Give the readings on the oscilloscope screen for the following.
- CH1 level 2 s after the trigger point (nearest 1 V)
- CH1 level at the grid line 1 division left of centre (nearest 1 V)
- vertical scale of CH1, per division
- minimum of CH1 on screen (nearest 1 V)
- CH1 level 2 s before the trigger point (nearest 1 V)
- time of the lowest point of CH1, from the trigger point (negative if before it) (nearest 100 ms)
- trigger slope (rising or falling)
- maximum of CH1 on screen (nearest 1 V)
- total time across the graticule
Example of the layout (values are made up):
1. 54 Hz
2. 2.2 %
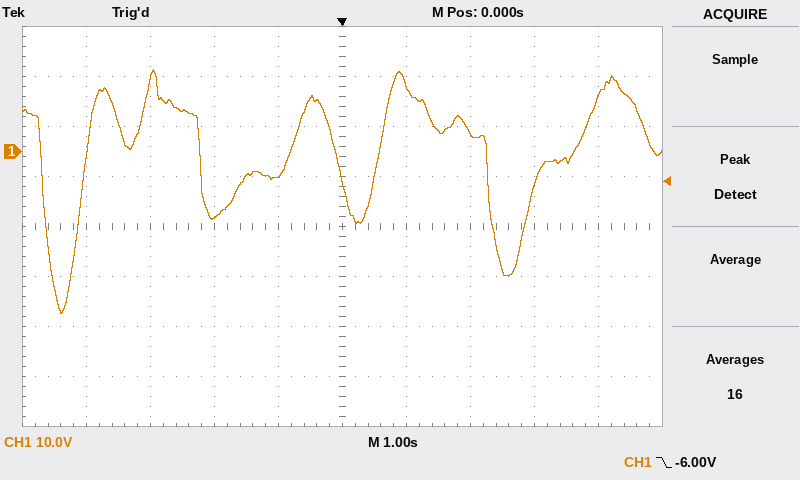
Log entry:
1. 4 V
2. -5 V
3. 10 V
4. -32 V
5. -13 V
6. -4.4 s
7. falling
8. 16 V
9. 10 s
